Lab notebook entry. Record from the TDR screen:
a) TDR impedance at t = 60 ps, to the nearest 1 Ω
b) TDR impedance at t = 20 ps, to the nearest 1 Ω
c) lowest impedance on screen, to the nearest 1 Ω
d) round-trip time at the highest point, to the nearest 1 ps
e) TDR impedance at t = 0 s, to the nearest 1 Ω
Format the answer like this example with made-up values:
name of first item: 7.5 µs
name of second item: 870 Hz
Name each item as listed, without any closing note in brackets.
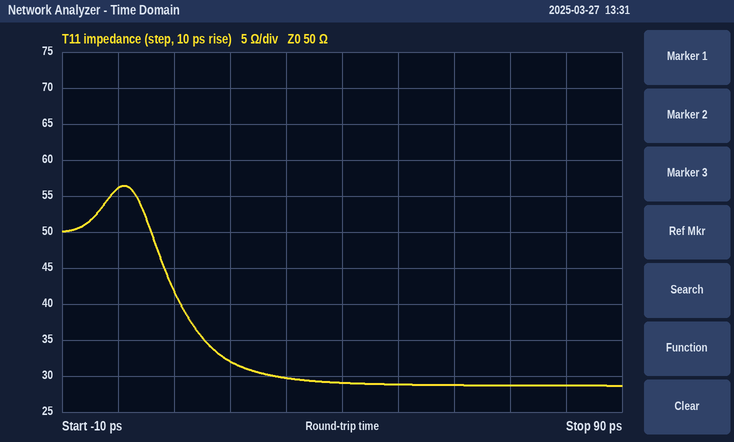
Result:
TDR impedance at t = 60 ps, to the nearest 1 Ω: 29 Ω
TDR impedance at t = 20 ps, to the nearest 1 Ω: 32 Ω
lowest impedance on screen, to the nearest 1 Ω: 29 Ω
round-trip time at the highest point, to the nearest 1 ps: 1 ps
TDR impedance at t = 0 s, to the nearest 1 Ω: 56 Ω
